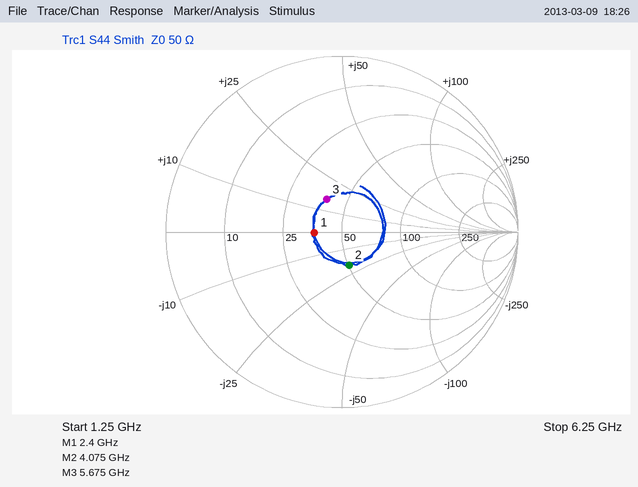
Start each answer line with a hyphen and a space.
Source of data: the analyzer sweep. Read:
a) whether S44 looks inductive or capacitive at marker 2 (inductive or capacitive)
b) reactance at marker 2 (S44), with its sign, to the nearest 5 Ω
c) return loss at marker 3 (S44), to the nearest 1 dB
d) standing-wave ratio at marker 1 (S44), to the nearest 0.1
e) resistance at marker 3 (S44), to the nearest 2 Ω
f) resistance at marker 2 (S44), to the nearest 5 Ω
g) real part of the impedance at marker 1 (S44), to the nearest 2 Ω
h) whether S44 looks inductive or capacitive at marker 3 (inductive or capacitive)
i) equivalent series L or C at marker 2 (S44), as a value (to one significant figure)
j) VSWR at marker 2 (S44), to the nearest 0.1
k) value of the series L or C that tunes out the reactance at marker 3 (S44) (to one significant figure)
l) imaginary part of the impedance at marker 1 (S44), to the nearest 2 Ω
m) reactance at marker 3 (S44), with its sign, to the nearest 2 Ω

- capacitive
- -20 Ω
- 14 dB
- 1.4
- 40 Ω
- 50 Ω
- 36 Ω
- inductive
- 2 pF
- 1.5
- 2 pF
- 0 Ω
- +16 Ω
